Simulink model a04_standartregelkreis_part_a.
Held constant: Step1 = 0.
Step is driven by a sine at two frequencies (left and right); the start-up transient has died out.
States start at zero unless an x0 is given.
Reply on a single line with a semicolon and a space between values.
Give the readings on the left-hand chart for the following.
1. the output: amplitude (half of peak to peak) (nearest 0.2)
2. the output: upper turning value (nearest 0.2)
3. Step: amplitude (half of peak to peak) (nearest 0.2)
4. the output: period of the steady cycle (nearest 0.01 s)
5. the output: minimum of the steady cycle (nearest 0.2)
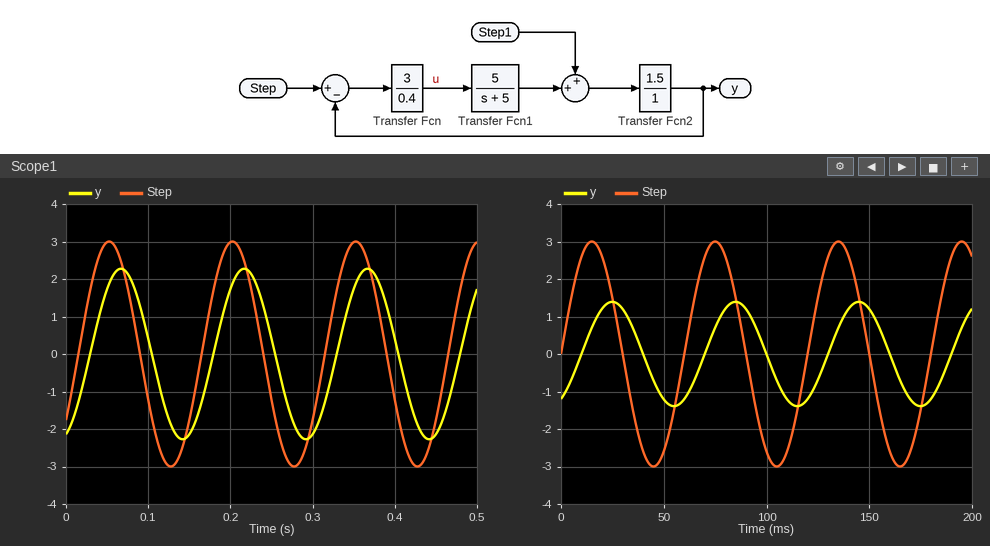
2.2; 2.2; 3.0; 0.15 s; -2.2
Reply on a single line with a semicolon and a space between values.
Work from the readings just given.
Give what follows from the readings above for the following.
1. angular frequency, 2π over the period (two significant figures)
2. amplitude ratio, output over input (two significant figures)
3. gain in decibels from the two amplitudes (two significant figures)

42 rad/s; 0.73; -2.7 dB
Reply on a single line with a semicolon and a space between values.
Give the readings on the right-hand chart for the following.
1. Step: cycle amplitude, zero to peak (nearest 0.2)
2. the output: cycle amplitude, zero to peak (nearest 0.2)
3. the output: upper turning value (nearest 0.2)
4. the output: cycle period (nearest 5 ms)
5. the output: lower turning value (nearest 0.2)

3.0; 1.4; 1.4; 60 ms; -1.4
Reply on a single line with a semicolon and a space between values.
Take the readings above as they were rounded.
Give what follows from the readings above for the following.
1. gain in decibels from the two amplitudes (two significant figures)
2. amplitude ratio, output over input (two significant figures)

-6.6 dB; 0.47
